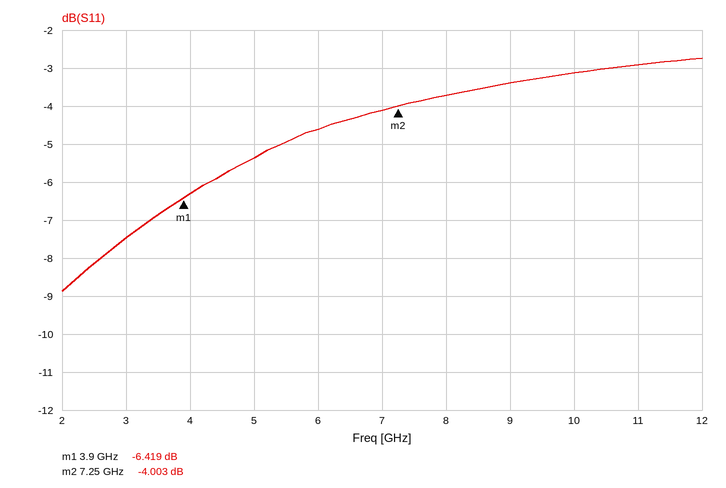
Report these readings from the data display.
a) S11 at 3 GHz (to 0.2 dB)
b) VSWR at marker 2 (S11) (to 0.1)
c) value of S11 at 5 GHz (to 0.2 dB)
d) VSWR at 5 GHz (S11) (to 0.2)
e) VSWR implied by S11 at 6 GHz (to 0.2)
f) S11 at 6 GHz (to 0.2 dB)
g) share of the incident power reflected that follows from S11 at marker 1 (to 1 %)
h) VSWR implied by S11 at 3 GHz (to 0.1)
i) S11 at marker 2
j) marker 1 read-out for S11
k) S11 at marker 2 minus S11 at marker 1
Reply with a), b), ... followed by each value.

a) -7.4 dB
b) 4.4
c) -5.4 dB
d) 3.4
e) 3.8
f) -4.6 dB
g) 23 %
h) 2.5
i) -4.003 dB
j) -6.419 dB
k) 2.416 dB
